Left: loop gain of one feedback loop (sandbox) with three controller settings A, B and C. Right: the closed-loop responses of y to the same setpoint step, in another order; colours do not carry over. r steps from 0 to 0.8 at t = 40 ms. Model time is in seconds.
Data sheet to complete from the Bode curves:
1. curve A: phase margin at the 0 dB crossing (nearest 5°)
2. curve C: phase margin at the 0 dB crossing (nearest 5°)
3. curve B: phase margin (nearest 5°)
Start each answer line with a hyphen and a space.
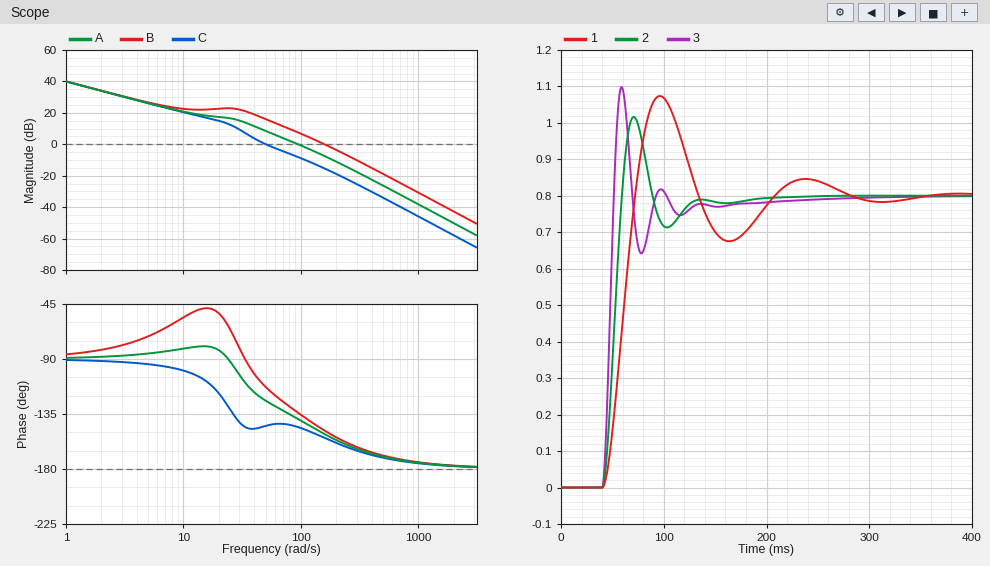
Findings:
- 40°
- 35°
- 30°
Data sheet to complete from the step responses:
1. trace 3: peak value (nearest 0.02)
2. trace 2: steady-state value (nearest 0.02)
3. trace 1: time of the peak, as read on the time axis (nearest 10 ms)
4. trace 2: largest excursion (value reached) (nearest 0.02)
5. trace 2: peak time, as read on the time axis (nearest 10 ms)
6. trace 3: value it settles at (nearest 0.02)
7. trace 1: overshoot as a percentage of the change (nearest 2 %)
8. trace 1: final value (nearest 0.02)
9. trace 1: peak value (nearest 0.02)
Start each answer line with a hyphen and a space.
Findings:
- 1.10
- 0.80
- 100 ms
- 1.02
- 70 ms
- 0.80
- 34 %
- 0.80
- 1.08
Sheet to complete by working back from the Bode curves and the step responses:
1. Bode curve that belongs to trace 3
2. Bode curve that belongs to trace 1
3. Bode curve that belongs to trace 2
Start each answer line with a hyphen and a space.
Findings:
- B
- C
- A
